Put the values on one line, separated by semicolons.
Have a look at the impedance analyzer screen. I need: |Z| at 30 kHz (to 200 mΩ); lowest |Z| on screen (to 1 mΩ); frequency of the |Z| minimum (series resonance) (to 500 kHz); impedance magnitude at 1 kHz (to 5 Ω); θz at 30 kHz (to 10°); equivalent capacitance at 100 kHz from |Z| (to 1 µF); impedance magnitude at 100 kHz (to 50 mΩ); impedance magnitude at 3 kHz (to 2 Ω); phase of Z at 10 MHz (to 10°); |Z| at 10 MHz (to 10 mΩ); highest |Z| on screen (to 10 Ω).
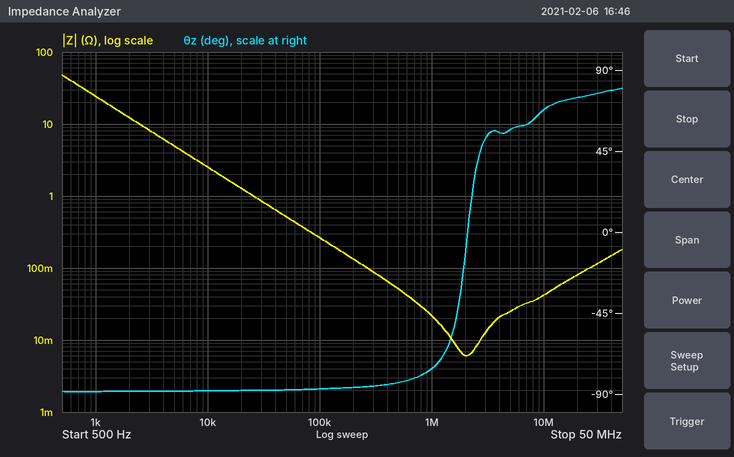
800 mΩ; 6 mΩ; 2.0 MHz; 25 Ω; -90°; 6 µF; 250 mΩ; 8 Ω; 70°; 40 mΩ; 50 Ω
